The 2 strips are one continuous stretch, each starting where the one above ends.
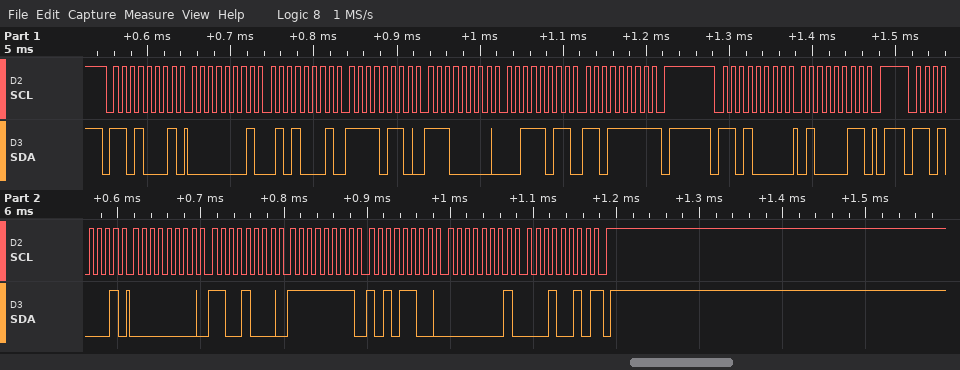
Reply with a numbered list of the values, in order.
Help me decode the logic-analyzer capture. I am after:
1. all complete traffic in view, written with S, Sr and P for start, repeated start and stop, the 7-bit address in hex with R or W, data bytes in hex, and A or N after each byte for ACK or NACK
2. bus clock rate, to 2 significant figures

1. S 68R A 01 A 51 A F6 A E0 A 3B A DF N P S 68W A 43 A P S 68R A 00 A C8 A FF A AC A 01 A 12 N P
2. 100 kHz
